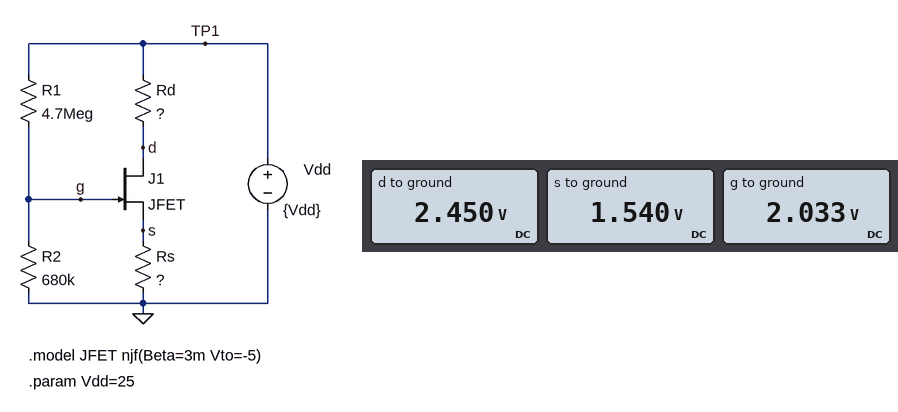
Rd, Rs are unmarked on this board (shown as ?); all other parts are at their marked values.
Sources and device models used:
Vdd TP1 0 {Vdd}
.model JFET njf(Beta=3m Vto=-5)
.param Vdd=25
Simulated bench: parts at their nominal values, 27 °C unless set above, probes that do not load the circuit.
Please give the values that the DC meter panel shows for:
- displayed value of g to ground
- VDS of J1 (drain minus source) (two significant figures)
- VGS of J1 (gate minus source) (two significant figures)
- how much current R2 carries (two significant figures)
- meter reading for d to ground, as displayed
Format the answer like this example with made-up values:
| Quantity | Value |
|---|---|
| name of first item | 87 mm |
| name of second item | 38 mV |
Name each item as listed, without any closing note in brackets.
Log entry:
| Quantity | Value |
|---|---|
| displayed value of g to ground | 2.033 V |
| VDS of J1 (drain minus source) | 910 mV |
| VGS of J1 (gate minus source) | 490 mV |
| how much current R2 carries | 3.0 µA |
| meter reading for d to ground, as displayed | 2.450 V |
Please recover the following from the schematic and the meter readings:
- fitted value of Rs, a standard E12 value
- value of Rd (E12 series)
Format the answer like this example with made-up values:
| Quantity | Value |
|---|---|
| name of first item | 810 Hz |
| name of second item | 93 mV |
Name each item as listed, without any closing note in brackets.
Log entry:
| Quantity | Value |
|---|---|
| fitted value of Rs, a standard E12 value | 56 Ω |
| value of Rd | 820 Ω |
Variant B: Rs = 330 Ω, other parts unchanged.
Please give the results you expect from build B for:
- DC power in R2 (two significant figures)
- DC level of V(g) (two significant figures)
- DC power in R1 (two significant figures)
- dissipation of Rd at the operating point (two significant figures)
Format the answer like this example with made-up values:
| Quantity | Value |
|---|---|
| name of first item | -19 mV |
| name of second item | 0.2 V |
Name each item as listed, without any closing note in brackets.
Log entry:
| Quantity | Value |
|---|---|
| DC power in R2 | 15 µW |
| DC level of V(g) | 3.2 V |
| DC power in R1 | 100 µW |
| dissipation of Rd at the operating point | 250 mW |
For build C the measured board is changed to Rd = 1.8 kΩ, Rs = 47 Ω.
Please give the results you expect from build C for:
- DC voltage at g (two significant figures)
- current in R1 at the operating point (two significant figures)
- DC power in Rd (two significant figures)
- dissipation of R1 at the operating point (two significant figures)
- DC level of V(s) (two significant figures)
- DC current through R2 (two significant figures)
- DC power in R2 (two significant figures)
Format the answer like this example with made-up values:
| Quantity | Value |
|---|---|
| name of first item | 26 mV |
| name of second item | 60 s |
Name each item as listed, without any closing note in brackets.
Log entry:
| Quantity | Value |
|---|---|
| DC voltage at g | 1.1 V |
| current in R1 at the operating point | 5.1 µA |
| DC power in Rd | 320 mW |
| dissipation of R1 at the operating point | 120 µW |
| DC level of V(s) | 630 mV |
| DC current through R2 | 1.7 µA |
| DC power in R2 | 1.9 µW |
